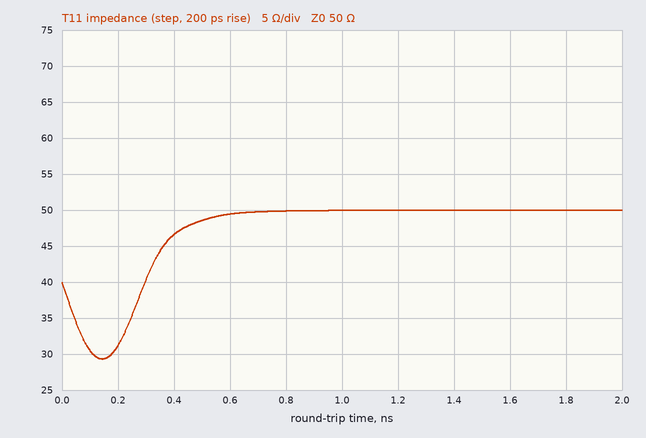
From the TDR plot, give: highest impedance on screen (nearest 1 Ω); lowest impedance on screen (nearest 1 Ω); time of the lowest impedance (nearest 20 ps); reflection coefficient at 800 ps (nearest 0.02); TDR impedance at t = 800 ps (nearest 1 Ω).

50 Ω
29 Ω
140 ps
0.00
50 Ω
